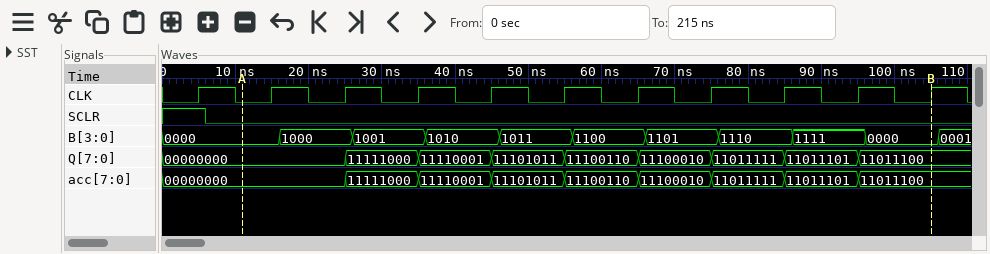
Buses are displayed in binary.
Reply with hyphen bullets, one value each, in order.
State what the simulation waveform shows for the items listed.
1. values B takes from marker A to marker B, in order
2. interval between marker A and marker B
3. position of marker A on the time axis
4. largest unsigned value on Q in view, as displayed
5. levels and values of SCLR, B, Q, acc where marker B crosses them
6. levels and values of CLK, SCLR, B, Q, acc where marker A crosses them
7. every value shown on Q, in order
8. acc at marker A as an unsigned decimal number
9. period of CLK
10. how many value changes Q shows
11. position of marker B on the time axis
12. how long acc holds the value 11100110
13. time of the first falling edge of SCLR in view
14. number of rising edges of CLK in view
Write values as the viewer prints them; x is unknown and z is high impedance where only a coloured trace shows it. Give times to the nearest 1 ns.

- 0000, 1000, 1001, 1010, 1011, 1100, 1101, 1110, 1111, 0000
- 94 ns
- 11 ns
- 11111000
- SCLR=0, B=0000, Q=11011100, acc=11011100
- CLK=0, SCLR=0, B=0000, Q=00000000, acc=00000000
- 00000000, 11111000, 11110001, 11101011, 11100110, 11100010, 11011111, 11011101, 11011100
- 0
- 10 ns
- 8
- 105 ns
- 10 ns
- 6 ns
- 11
